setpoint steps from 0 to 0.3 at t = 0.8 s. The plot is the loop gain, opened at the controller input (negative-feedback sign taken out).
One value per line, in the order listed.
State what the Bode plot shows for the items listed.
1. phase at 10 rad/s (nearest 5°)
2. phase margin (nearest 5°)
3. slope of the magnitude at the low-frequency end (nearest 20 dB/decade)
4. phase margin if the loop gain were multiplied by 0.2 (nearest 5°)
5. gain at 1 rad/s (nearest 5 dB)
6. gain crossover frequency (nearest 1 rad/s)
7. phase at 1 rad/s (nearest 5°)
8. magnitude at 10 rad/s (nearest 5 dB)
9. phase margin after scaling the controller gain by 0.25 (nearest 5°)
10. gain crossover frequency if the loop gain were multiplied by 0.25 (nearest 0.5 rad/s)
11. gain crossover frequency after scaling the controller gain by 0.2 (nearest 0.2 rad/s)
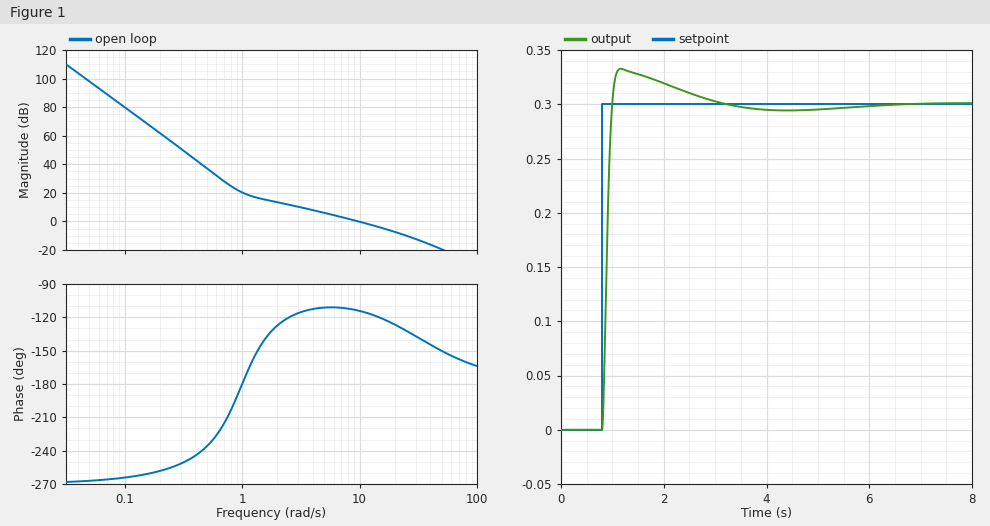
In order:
-115°
65°
-60 dB/decade
50°
20 dB
10 rad/s
-180°
0 dB
60°
2.5 rad/s
1.8 rad/s
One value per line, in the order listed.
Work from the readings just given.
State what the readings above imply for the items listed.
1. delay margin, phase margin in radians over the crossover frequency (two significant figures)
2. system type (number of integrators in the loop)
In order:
0.11 s
3
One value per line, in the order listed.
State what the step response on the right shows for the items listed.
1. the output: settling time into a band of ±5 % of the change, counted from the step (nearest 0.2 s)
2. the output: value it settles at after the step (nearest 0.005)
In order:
1.4 s
0.300
